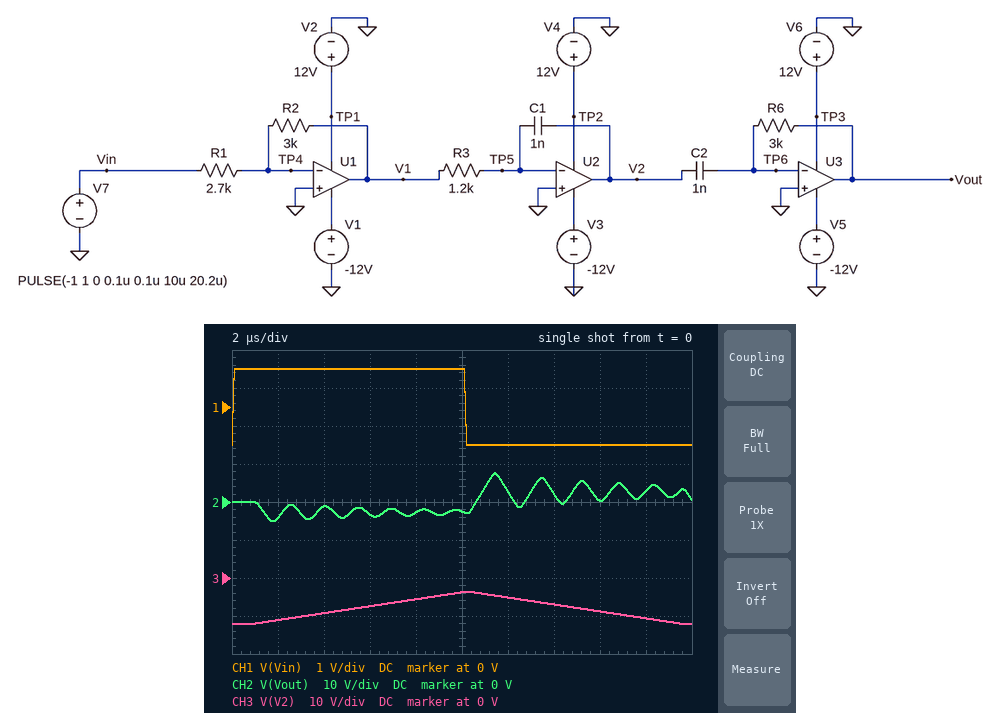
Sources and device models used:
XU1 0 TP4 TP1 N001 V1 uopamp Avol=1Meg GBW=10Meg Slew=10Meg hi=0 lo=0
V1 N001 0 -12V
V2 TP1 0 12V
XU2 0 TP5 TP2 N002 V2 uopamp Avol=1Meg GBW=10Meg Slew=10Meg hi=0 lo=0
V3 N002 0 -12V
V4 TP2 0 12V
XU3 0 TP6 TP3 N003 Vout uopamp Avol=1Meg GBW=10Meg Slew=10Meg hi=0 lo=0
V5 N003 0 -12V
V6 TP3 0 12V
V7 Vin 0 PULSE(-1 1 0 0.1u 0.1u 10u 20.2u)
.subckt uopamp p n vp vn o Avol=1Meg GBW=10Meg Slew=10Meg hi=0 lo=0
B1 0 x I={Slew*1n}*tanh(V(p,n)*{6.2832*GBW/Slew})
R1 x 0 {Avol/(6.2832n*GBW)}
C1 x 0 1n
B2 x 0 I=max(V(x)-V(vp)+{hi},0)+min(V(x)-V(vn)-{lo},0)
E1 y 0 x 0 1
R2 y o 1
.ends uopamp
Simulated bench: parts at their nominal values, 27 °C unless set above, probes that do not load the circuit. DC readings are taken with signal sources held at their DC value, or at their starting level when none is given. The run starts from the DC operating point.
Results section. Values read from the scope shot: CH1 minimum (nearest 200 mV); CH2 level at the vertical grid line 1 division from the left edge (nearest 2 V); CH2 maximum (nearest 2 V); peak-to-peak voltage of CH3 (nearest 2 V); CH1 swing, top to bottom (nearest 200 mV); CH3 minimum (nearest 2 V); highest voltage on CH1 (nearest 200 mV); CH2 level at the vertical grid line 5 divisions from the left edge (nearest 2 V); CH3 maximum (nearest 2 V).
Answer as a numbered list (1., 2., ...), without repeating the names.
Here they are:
1. -1.0 V
2. -4 V
3. 8 V
4. 8 V
5. 2.0 V
6. -12 V
7. 1.0 V
8. -2 V
9. -4 V
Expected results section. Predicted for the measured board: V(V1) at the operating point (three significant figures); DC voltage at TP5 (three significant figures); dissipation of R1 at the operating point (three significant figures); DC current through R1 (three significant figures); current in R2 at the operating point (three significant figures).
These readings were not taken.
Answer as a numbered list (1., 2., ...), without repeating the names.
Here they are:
1. 1.11 V
2. 1.11 V
3. 370 µW
4. 370 µA
5. 370 µA
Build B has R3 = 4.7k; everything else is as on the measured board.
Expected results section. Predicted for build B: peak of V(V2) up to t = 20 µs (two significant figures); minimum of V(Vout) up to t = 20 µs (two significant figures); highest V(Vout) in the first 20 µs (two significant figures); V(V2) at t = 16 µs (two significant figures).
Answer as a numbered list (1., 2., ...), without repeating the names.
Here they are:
1. -10 V
2. -1.3 V
3. 1.7 V
4. -12 V
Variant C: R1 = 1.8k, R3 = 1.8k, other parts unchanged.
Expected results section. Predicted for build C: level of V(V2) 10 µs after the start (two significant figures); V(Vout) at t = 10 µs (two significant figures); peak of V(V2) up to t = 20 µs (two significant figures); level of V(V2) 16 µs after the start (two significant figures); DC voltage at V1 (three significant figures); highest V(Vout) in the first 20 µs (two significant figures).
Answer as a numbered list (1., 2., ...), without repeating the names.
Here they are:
1. -4.2 V
2. -2.4 V
3. -4.0 V
4. -9.1 V
5. 1.67 V
6. 6.6 V
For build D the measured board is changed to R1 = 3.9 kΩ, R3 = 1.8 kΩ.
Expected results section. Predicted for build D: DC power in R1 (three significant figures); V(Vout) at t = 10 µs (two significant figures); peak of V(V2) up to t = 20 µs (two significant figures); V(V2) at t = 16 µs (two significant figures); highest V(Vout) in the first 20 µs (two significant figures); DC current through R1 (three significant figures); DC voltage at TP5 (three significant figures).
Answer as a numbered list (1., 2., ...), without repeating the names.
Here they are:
1. 256 µW
2. -1.2 V
3. -8.3 V
4. -11 V
5. 3.6 V
6. 256 µA
7. 769 mV
